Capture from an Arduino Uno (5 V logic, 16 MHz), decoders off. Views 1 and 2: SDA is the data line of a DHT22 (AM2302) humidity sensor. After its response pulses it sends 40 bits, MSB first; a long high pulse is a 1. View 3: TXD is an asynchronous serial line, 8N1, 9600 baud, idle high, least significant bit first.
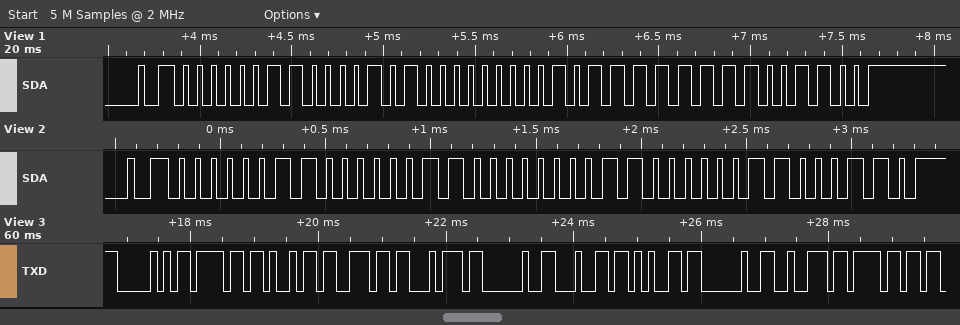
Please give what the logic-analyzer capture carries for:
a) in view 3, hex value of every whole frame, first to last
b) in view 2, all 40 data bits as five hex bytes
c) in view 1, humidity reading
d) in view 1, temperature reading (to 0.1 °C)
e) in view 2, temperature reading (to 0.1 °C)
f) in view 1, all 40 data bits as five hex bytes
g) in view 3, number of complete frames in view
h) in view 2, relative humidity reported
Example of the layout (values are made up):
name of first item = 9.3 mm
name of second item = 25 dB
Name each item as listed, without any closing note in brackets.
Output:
in view 3, hex value of every whole frame, first to last = 50 6F 69 6E 74 20 64 65 20 72 6F
in view 2, all 40 data bits as five hex bytes = 03 03 00 C0 C6
in view 1, humidity reading = 77.8 %
in view 1, temperature reading = 19.1 °C
in view 2, temperature reading = 19.2 °C
in view 1, all 40 data bits as five hex bytes = 03 0A 00 BF CC
in view 3, number of complete frames in view = 11
in view 2, relative humidity reported = 77.1 %
